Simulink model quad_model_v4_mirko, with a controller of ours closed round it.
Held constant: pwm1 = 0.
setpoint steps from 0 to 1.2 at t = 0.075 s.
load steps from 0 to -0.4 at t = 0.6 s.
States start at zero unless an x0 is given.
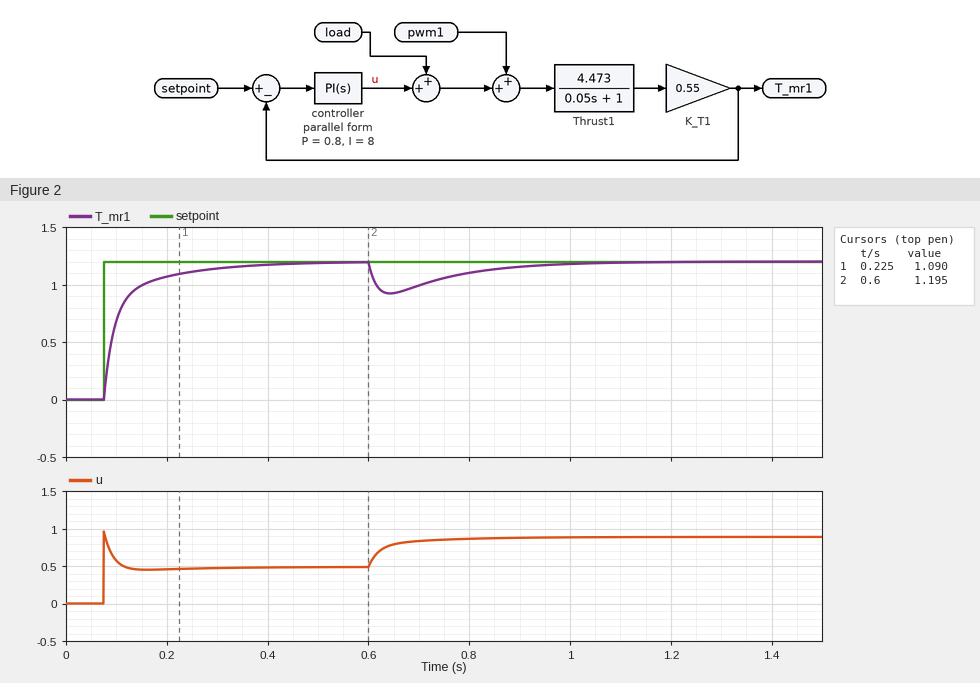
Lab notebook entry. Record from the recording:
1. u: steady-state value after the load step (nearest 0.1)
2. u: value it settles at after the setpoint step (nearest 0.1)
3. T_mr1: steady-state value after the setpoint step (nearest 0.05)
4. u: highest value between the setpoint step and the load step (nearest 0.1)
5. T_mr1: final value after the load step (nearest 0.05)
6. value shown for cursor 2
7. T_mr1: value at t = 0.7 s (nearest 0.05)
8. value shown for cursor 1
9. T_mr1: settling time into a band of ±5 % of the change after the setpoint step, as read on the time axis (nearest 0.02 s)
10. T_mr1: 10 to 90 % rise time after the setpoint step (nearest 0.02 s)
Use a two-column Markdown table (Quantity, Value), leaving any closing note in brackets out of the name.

| Quantity | Value |
|---|---|
| u: steady-state value after the load step | 0.9 |
| u: value it settles at after the setpoint step | 0.5 |
| T_mr1: steady-state value after the setpoint step | 1.20 |
| u: highest value between the setpoint step and the load step | 1.0 |
| T_mr1: final value after the load step | 1.20 |
| value shown for cursor 2 | 1.195 |
| T_mr1: value at t = 0.7 s | 1.00 |
| value shown for cursor 1 | 1.090 |
| T_mr1: settling time into a band of ±5 % of the change after the setpoint step, as read on the time axis | 0.30 s |
| T_mr1: 10 to 90 % rise time after the setpoint step | 0.14 s |
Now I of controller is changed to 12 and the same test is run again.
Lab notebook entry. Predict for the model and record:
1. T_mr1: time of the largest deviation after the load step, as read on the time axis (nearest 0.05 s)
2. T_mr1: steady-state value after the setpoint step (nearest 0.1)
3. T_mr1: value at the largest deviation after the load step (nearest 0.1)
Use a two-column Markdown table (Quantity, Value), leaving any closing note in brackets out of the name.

| Quantity | Value |
|---|---|
| T_mr1: time of the largest deviation after the load step, as read on the time axis | 0.65 s |
| T_mr1: steady-state value after the setpoint step | 1.2 |
| T_mr1: value at the largest deviation after the load step | 0.9 |
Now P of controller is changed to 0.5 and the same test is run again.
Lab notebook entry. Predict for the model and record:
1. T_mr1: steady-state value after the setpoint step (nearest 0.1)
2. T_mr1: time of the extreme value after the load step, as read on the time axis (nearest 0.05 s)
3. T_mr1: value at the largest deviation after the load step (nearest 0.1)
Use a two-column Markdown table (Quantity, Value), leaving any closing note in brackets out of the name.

| Quantity | Value |
|---|---|
| T_mr1: steady-state value after the setpoint step | 1.2 |
| T_mr1: time of the extreme value after the load step, as read on the time axis | 0.65 s |
| T_mr1: value at the largest deviation after the load step | 0.9 |
